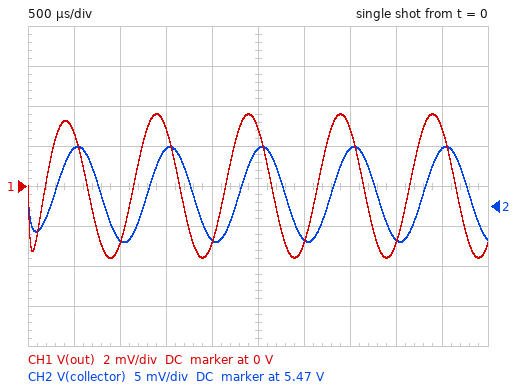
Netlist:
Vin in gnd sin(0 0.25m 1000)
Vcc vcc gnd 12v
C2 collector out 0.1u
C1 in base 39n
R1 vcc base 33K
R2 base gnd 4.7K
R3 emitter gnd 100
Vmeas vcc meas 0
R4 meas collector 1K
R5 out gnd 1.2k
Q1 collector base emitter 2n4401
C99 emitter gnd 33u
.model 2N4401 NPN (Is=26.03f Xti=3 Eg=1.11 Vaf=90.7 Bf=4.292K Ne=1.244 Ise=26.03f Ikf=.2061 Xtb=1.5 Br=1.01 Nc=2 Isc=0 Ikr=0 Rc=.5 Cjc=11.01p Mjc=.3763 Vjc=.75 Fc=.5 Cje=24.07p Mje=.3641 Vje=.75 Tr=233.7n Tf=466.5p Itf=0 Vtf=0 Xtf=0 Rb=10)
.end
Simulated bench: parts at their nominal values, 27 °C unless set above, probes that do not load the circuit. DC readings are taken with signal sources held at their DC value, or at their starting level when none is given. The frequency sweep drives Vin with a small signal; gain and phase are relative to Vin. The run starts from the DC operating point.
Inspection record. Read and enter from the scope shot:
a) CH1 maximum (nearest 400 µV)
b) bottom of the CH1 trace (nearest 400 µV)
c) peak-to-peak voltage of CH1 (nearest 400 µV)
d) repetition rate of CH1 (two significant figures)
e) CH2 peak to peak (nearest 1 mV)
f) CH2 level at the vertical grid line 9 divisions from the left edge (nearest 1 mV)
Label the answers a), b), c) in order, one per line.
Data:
a) 3.6 mV
b) -3.6 mV
c) 7.2 mV
d) 1.0 kHz
e) 12 mV
f) 5.477 V
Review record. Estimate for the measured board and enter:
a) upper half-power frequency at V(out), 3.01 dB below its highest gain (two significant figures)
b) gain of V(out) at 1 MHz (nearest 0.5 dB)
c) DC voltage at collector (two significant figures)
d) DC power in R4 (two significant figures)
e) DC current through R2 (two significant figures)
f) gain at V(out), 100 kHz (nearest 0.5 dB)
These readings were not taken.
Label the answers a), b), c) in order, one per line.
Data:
a) 15 MHz
b) 42.0 dB
c) 5.5 V
d) 43 mW
e) 280 µA
f) 42.0 dB
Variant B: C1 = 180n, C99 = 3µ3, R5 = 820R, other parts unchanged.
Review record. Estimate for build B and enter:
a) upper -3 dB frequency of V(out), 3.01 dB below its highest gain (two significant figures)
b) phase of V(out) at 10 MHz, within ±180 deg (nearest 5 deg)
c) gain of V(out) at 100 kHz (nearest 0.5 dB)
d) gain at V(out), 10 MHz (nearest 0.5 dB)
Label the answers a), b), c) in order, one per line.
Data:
a) 17 MHz
b) 150 deg
c) 40.5 dB
d) 39.0 dB
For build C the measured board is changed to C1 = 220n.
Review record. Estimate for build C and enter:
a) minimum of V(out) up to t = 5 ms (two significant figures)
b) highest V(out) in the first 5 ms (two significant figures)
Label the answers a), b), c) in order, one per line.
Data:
a) -11 mV
b) 11 mV
